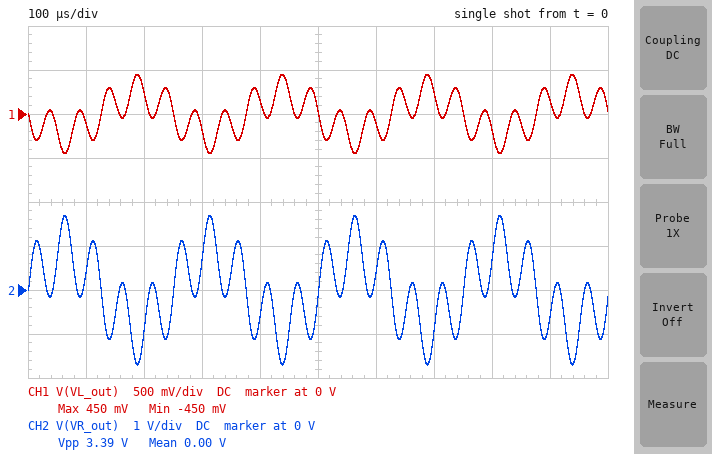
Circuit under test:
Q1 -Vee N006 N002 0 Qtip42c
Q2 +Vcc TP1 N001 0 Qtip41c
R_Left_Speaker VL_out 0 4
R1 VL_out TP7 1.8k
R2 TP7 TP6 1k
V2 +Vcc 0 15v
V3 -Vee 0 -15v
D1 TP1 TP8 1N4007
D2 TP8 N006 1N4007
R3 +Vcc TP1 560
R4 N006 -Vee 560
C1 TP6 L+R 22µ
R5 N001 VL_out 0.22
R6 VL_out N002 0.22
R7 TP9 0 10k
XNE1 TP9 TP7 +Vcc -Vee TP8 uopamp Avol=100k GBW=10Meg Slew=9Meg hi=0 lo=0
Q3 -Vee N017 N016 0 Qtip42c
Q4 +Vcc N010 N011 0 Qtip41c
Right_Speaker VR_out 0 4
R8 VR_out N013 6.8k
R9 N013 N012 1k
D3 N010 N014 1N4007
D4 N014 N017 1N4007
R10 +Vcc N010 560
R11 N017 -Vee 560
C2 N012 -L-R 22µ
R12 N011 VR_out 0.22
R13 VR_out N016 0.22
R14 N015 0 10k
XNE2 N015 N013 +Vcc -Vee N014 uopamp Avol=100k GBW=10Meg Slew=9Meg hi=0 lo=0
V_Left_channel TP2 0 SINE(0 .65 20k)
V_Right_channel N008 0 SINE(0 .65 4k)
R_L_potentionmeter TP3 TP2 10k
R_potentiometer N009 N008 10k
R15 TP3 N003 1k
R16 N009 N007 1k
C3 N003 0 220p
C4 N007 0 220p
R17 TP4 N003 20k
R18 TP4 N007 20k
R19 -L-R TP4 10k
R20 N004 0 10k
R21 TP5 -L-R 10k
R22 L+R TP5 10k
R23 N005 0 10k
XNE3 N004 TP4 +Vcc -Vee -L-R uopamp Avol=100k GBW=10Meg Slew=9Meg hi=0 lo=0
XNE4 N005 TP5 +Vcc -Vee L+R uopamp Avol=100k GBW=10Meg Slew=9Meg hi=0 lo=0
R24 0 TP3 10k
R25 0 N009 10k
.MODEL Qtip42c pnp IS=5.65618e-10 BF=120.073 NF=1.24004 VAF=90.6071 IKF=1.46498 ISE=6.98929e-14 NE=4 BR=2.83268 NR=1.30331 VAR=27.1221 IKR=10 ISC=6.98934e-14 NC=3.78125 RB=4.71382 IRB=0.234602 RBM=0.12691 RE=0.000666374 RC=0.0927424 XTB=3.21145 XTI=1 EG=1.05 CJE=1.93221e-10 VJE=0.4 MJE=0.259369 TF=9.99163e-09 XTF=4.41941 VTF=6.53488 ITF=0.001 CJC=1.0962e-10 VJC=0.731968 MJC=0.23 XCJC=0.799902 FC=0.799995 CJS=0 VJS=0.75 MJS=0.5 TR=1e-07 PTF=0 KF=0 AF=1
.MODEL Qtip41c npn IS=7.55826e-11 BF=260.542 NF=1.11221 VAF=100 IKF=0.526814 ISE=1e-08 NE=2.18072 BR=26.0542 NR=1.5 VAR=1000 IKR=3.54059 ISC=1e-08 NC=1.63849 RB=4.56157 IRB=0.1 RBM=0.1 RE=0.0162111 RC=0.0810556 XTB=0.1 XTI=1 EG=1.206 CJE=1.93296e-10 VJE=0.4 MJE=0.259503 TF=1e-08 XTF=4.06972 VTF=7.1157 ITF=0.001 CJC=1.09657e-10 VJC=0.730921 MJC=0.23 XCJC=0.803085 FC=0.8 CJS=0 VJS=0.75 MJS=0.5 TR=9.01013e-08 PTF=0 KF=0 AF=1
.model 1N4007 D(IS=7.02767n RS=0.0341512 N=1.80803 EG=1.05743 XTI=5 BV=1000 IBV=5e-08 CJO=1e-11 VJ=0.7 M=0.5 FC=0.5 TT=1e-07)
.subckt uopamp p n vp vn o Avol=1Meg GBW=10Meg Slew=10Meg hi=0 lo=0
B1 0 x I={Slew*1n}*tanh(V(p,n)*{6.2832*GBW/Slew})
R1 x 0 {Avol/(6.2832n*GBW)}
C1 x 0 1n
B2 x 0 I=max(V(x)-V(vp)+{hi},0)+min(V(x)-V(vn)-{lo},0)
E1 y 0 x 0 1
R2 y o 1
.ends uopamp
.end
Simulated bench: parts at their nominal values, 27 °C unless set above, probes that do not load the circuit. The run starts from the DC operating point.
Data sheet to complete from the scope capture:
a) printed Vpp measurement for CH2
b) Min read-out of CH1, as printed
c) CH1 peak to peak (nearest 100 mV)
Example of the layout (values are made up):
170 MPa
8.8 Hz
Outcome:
3.39 V
-450 mV
900 mV
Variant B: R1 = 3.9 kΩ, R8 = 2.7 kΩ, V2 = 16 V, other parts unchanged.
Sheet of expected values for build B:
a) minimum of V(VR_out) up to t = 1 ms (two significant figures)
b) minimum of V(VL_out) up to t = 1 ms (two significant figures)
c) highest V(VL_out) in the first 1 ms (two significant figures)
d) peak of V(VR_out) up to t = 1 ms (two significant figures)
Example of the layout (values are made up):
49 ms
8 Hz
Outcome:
-670 mV
-970 mV
970 mV
670 mV
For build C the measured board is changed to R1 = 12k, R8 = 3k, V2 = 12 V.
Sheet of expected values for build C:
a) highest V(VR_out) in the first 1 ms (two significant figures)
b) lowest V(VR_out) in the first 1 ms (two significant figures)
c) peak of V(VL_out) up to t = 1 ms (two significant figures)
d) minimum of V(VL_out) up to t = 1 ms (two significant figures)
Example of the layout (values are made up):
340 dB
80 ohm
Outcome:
750 mV
-750 mV
3.0 V
-3.0 V
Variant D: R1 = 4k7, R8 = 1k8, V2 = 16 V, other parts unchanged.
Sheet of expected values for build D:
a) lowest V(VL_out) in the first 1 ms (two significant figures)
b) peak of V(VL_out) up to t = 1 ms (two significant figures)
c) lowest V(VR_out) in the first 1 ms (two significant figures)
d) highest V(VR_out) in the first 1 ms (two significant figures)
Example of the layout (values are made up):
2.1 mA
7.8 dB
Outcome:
-1.2 V
1.2 V
-450 mV
450 mV
